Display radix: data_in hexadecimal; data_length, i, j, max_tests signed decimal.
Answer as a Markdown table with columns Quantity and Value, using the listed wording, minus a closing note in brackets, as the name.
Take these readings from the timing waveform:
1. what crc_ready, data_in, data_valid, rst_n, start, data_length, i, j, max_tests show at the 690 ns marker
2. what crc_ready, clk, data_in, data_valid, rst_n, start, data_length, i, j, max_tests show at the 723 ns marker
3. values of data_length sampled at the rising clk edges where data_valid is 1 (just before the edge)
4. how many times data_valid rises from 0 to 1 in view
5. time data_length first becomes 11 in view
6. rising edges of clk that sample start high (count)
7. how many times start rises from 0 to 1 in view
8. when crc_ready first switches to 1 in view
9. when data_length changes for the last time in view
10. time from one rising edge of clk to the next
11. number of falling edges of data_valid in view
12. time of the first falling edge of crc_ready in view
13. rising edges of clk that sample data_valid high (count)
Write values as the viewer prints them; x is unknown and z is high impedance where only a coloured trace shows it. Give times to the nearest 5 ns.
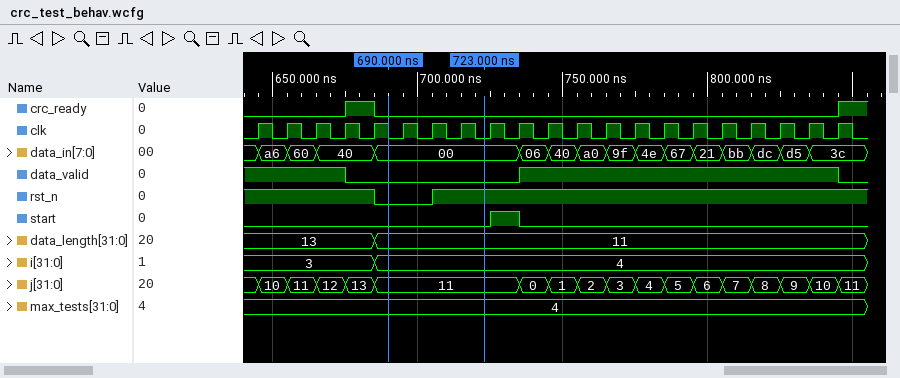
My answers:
| Quantity | Value |
|---|---|
| what crc_ready, data_in, data_valid, rst_n, start, data_length, i, j, max_tests show at the 690 ns marker | crc_ready=0, data_in=00, data_valid=0, rst_n=0, start=0, data_length=11, i=4, j=11, max_tests=4 |
| what crc_ready, clk, data_in, data_valid, rst_n, start, data_length, i, j, max_tests show at the 723 ns marker | crc_ready=0, clk=0, data_in=00, data_valid=0, rst_n=1, start=0, data_length=11, i=4, j=11, max_tests=4 |
| values of data_length sampled at the rising clk edges where data_valid is 1 | 13, 13, 13, 13, 11, 11, 11, 11, 11, 11, 11, 11, 11, 11, 11 |
| how many times data_valid rises from 0 to 1 in view | 1 |
| time data_length first becomes 11 in view | 685 ns |
| rising edges of clk that sample start high | 1 |
| how many times start rises from 0 to 1 in view | 1 |
| when crc_ready first switches to 1 in view | 675 ns |
| when data_length changes for the last time in view | 685 ns |
| time from one rising edge of clk to the next | 10 ns |
| number of falling edges of data_valid in view | 2 |
| time of the first falling edge of crc_ready in view | 685 ns |
| rising edges of clk that sample data_valid high | 15 |
